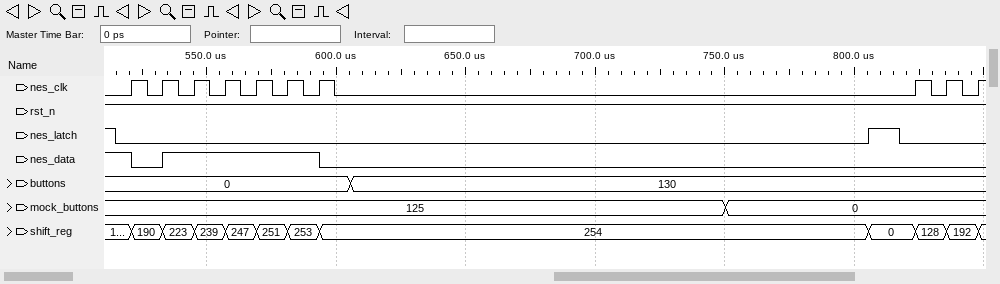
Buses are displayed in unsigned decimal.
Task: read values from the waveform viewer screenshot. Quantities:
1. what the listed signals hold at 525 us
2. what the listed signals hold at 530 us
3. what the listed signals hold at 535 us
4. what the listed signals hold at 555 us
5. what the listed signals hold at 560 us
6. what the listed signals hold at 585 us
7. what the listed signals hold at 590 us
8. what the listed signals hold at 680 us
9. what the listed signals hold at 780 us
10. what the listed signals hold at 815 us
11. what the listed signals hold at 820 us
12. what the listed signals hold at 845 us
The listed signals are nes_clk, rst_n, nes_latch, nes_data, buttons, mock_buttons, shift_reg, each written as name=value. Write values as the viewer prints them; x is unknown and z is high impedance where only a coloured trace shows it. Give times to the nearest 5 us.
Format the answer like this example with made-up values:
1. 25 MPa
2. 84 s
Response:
1. nes_clk=1, rst_n=1, nes_latch=0, nes_data=0, buttons=0, mock_buttons=125, shift_reg=190
2. nes_clk=0, rst_n=1, nes_latch=0, nes_data=0, buttons=0, mock_buttons=125, shift_reg=190
3. nes_clk=1, rst_n=1, nes_latch=0, nes_data=1, buttons=0, mock_buttons=125, shift_reg=223
4. nes_clk=0, rst_n=1, nes_latch=0, nes_data=1, buttons=0, mock_buttons=125, shift_reg=239
5. nes_clk=1, rst_n=1, nes_latch=0, nes_data=1, buttons=0, mock_buttons=125, shift_reg=247
6. nes_clk=1, rst_n=1, nes_latch=0, nes_data=1, buttons=0, mock_buttons=125, shift_reg=253
7. nes_clk=0, rst_n=1, nes_latch=0, nes_data=1, buttons=0, mock_buttons=125, shift_reg=253
8. nes_clk=0, rst_n=1, nes_latch=0, nes_data=0, buttons=130, mock_buttons=125, shift_reg=254
9. nes_clk=0, rst_n=1, nes_latch=0, nes_data=0, buttons=130, mock_buttons=0, shift_reg=254
10. nes_clk=0, rst_n=1, nes_latch=1, nes_data=0, buttons=130, mock_buttons=0, shift_reg=0
11. nes_clk=0, rst_n=1, nes_latch=0, nes_data=0, buttons=130, mock_buttons=0, shift_reg=0
12. nes_clk=0, rst_n=1, nes_latch=0, nes_data=0, buttons=130, mock_buttons=0, shift_reg=192
